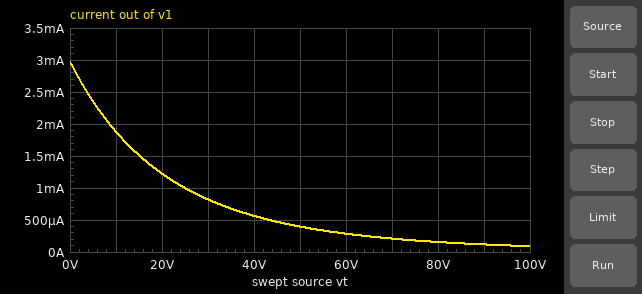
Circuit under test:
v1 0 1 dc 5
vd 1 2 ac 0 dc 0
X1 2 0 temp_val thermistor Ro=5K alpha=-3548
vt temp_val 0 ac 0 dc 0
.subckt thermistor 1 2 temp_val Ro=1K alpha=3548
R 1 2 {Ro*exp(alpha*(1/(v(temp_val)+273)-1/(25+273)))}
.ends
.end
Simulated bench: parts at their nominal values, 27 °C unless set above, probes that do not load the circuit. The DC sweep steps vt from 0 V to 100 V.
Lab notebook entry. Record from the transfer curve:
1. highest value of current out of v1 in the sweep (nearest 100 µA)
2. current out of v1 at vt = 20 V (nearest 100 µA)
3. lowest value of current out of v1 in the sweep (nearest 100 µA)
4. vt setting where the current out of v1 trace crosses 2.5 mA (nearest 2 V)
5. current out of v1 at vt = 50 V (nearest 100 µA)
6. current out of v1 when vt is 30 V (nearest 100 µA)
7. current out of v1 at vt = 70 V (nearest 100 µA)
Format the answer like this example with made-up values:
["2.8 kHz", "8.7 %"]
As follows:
["3.0 mA", "1.2 mA", "100 µA", "4 V", "400 µA", "800 µA", "200 µA"]
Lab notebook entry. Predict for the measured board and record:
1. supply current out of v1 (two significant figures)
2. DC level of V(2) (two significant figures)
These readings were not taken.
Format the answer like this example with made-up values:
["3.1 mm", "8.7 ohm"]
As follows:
["3.0 mA", "-5.0 V"]
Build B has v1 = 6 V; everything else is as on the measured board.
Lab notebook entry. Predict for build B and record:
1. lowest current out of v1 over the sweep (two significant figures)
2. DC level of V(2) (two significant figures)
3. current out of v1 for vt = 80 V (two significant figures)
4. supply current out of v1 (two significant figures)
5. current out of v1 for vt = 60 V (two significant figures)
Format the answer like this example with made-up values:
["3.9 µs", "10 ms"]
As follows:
["110 µA", "-6.0 V", "190 µA", "3.6 mA", "340 µA"]
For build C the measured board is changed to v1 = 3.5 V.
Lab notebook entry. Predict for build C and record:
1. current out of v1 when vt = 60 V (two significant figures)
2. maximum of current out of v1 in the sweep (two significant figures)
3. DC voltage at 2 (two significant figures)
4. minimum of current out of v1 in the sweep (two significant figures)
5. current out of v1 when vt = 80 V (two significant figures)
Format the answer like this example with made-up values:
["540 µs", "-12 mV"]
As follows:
["200 µA", "2.1 mA", "-3.5 V", "64 µA", "110 µA"]
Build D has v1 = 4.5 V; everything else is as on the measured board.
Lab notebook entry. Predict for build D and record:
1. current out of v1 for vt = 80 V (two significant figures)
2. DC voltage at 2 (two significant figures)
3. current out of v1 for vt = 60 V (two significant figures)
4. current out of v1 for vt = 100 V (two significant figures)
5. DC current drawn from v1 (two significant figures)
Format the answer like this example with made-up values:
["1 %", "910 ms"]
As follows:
["140 µA", "-4.5 V", "260 µA", "82 µA", "2.7 mA"]
